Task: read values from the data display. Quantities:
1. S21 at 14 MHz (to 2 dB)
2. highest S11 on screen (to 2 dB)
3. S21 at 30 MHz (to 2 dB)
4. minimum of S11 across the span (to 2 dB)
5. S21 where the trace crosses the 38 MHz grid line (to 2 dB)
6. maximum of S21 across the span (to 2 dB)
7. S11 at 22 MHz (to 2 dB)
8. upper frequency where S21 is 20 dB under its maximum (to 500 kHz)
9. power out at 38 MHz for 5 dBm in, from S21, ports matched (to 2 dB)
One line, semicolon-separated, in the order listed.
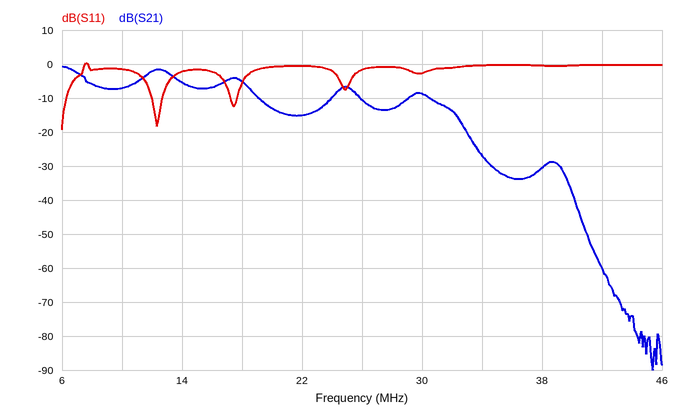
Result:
-6 dB; 0 dB; -8 dB; -20 dB; -30 dB; 0 dB; 0 dB; 33.0 MHz; -26 dBm
